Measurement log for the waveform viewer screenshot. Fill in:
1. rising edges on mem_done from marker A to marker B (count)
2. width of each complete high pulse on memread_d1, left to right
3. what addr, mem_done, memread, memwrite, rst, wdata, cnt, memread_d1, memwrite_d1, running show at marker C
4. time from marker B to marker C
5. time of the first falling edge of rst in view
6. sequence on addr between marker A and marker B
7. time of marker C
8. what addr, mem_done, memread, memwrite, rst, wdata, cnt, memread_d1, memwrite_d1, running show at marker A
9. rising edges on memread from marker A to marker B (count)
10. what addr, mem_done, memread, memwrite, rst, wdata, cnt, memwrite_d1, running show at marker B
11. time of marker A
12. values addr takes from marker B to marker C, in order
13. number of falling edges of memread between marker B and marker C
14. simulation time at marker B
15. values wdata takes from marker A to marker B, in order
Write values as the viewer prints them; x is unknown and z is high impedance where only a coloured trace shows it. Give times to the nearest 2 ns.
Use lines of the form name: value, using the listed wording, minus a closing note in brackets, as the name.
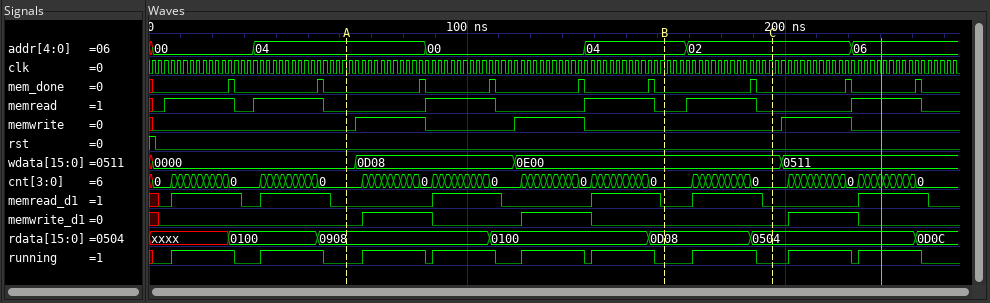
rising edges on mem_done from marker A to marker B: 4
width of each complete high pulse on memread_d1, left to right: 22 ns, 22 ns, 22 ns, 22 ns, 22 ns, 22 ns
what addr, mem_done, memread, memwrite, rst, wdata, cnt, memread_d1, memwrite_d1, running show at marker C: addr=02, mem_done=0, memread=0, memwrite=0, rst=0, wdata=0E00, cnt=0, memread_d1=0, memwrite_d1=0, running=0
time from marker B to marker C: 34 ns
time of the first falling edge of rst in view: 2 ns
sequence on addr between marker A and marker B: 04, 00, 04
time of marker C: 196 ns
what addr, mem_done, memread, memwrite, rst, wdata, cnt, memread_d1, memwrite_d1, running show at marker A: addr=04, mem_done=0, memread=0, memwrite=0, rst=0, wdata=0000, cnt=0, memread_d1=0, memwrite_d1=0, running=0
rising edges on memread from marker A to marker B: 2
what addr, mem_done, memread, memwrite, rst, wdata, cnt, memwrite_d1, running show at marker B: addr=04, mem_done=0, memread=0, memwrite=0, rst=0, wdata=0E00, cnt=0, memwrite_d1=0, running=0
time of marker A: 62 ns
values addr takes from marker B to marker C, in order: 04, 02
number of falling edges of memread between marker B and marker C: 1
simulation time at marker B: 162 ns
values wdata takes from marker A to marker B, in order: 0000, 0D08, 0E00
